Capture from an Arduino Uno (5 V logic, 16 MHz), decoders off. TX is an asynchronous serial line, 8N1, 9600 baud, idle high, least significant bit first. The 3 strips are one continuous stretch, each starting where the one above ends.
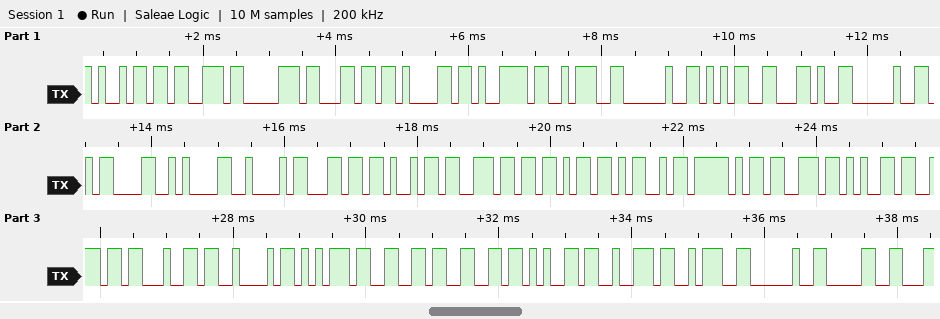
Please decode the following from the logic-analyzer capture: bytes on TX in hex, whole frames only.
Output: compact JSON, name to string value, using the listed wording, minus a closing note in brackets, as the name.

{"bytes on TX in hex, whole frames only": "69 73 70 6C 61 79 3A 20 35 2C 20 0D 0A 42 6C 69 6E 6B 4D 5F 73 65 6E 64 42 75 66 66 65 72 3A 20 30"}
